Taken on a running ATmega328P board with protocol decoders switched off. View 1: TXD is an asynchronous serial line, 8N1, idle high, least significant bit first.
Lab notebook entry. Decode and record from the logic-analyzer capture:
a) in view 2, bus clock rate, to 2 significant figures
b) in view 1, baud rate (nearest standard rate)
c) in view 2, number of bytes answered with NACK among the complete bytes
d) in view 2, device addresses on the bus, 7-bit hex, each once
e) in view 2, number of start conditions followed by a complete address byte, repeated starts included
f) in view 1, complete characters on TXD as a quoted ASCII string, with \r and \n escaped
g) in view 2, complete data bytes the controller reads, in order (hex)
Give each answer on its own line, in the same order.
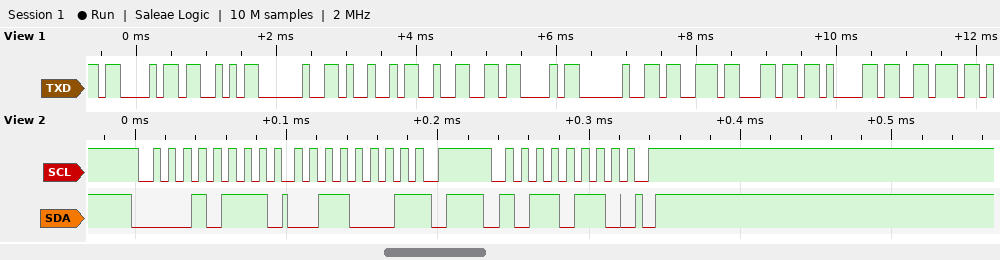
100 kHz
9600 baud
1
0x0B 0x5B
2
"CS I2C slav"
31
